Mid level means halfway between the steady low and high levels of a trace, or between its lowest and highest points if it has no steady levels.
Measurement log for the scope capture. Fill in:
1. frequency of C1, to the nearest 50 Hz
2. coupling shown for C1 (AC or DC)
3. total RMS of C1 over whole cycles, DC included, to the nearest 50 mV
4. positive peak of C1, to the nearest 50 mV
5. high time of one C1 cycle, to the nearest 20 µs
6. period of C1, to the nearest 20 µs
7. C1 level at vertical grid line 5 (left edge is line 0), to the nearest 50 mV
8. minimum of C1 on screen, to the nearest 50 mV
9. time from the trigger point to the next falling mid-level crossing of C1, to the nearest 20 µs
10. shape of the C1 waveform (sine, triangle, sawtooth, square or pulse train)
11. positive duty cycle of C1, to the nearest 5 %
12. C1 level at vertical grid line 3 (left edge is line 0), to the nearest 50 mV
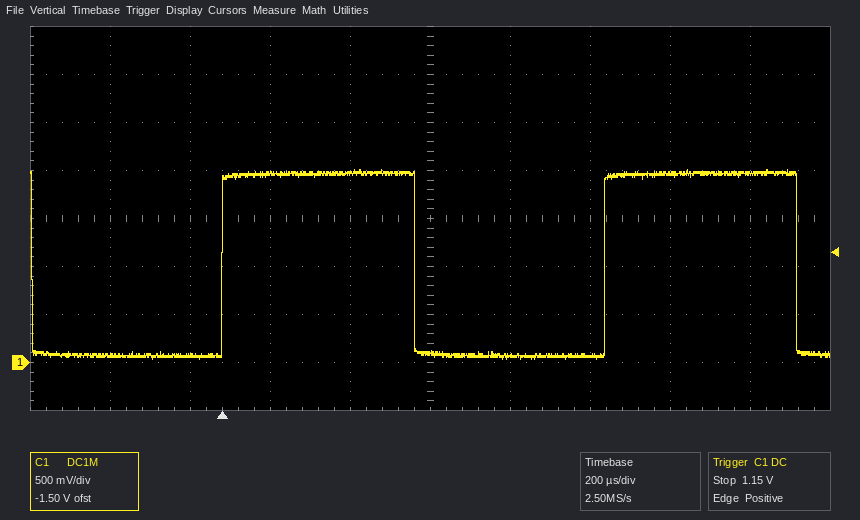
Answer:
1.05 kHz
DC
1.40 V
2.00 V
480 µs
960 µs
100 mV
50 mV
480 µs
square
50 %
1.95 V
